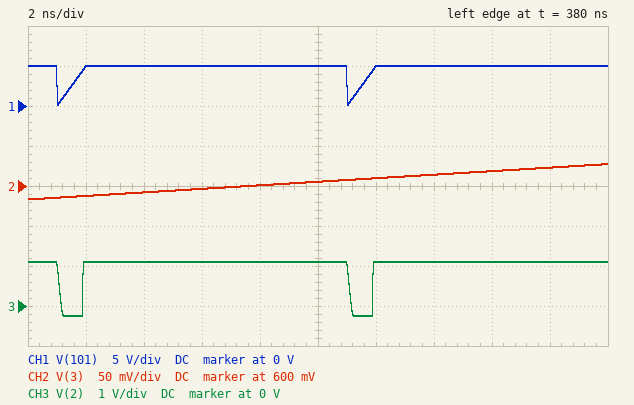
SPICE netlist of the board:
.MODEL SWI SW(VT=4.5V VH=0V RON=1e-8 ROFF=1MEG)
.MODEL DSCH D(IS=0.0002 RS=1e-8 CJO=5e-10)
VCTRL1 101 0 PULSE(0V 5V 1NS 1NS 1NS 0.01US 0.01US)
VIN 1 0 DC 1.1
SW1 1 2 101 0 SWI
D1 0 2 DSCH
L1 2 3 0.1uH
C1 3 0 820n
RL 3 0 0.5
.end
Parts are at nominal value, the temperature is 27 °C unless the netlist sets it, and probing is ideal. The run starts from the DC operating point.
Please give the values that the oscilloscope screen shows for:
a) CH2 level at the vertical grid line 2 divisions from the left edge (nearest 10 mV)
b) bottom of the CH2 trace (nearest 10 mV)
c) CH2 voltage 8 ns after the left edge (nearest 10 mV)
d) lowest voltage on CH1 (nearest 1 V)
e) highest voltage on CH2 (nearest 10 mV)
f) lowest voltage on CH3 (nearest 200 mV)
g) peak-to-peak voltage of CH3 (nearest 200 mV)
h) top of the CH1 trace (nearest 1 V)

590 mV
580 mV
600 mV
0 V
630 mV
-200 mV
1.4 V
5 V
